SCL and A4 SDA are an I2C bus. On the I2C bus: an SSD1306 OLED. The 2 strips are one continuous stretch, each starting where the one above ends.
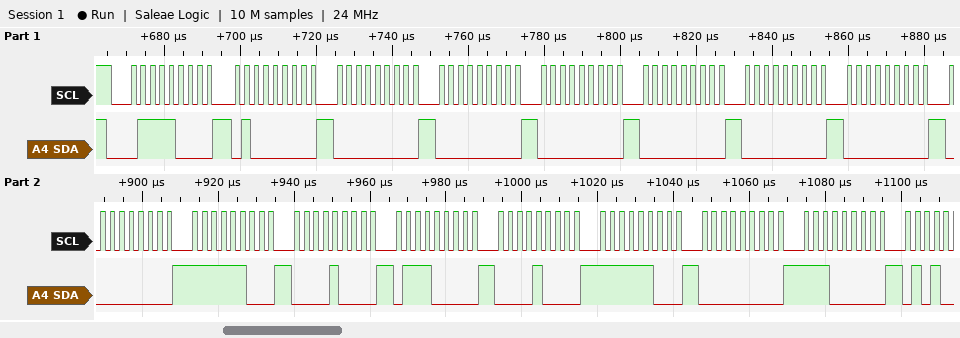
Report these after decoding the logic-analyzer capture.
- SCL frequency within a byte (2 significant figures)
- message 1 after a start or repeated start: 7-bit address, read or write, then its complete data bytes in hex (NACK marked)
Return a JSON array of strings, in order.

["400 kHz", "0x3C write: 40 00 00 00 00 00 00 00 FC 08 70 08 FC 00 E0"]
